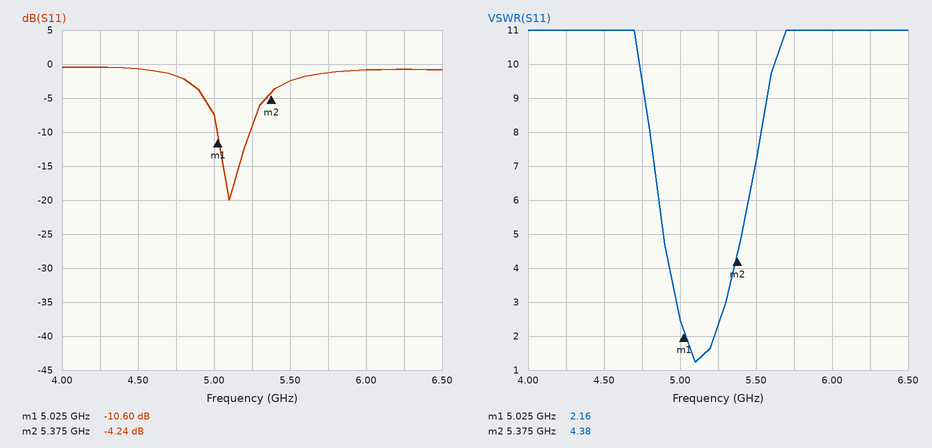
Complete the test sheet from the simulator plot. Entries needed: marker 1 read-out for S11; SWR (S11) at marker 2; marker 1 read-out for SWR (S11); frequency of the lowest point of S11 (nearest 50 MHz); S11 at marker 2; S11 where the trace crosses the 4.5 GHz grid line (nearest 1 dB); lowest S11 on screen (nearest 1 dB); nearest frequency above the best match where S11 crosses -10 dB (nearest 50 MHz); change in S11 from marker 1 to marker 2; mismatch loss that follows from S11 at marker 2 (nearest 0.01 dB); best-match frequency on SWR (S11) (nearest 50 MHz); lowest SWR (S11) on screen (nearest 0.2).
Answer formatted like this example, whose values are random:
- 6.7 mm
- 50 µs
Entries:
- -10.60 dB
- 4.38
- 2.16
- 5.10 GHz
- -4.24 dB
- -1 dB
- -20 dB
- 5.25 GHz
- 6.36 dB
- 2.05 dB
- 5.10 GHz
- 1.2
